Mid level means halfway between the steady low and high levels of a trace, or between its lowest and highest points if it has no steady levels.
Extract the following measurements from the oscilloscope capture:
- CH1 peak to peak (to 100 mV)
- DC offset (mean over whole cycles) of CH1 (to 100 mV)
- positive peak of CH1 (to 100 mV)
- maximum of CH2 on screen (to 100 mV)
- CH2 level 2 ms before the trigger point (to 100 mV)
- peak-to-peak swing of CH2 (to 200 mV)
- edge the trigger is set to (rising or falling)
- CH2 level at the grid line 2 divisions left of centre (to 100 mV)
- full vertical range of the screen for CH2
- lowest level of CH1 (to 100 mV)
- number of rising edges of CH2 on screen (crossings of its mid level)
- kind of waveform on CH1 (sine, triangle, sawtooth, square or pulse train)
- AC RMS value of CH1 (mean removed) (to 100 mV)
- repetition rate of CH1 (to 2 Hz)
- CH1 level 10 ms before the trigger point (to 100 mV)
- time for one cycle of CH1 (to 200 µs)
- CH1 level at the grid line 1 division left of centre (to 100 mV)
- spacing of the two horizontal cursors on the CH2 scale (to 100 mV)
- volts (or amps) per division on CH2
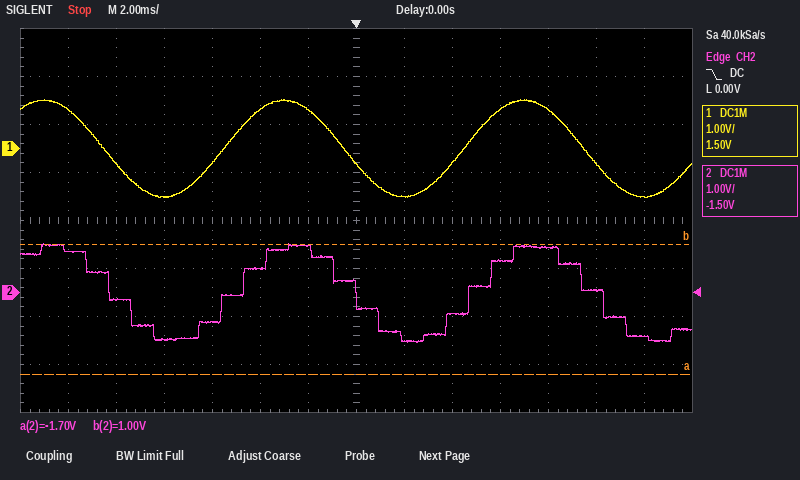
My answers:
2.0 V
0.0 V
1.0 V
1.0 V
1.0 V
2.0 V
falling
500 mV
8 V
-1.0 V
2
sine
700 mV
100 Hz
-300 mV
10.0 ms
800 mV
2.7 V
1 V
